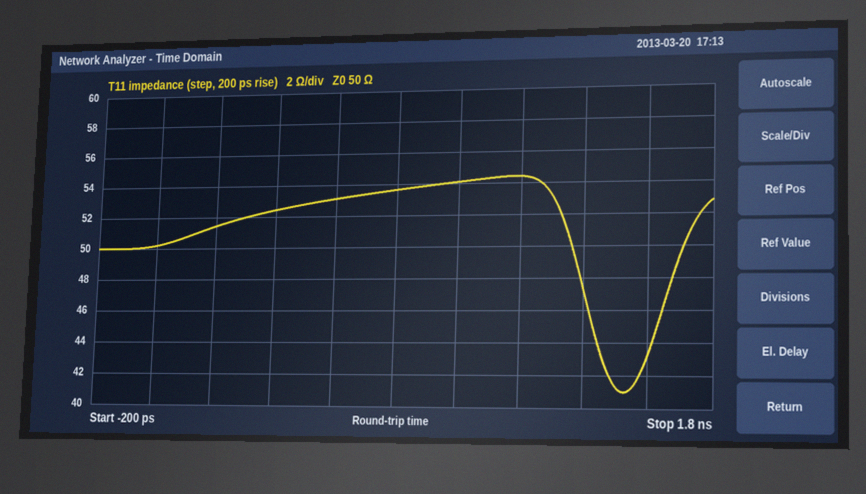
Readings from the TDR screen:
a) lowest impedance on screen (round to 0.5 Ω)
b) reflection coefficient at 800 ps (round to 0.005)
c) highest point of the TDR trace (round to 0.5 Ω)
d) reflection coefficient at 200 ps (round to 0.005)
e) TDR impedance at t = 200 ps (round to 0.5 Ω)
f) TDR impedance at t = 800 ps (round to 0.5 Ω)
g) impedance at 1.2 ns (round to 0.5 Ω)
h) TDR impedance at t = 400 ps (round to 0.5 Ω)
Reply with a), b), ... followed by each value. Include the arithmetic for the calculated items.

a) 41.0 Ω
b) (53.5 − 50)/(53.5 + 50) ≈ +0.0338, so +0.035 to the nearest 0.005
c) 54.5 Ω
d) (51.5 − 50)/(51.5 + 50) ≈ +0.015
e) 51.5 Ω
f) 53.5 Ω
g) 54.5 Ω
h) 52.5 Ω
